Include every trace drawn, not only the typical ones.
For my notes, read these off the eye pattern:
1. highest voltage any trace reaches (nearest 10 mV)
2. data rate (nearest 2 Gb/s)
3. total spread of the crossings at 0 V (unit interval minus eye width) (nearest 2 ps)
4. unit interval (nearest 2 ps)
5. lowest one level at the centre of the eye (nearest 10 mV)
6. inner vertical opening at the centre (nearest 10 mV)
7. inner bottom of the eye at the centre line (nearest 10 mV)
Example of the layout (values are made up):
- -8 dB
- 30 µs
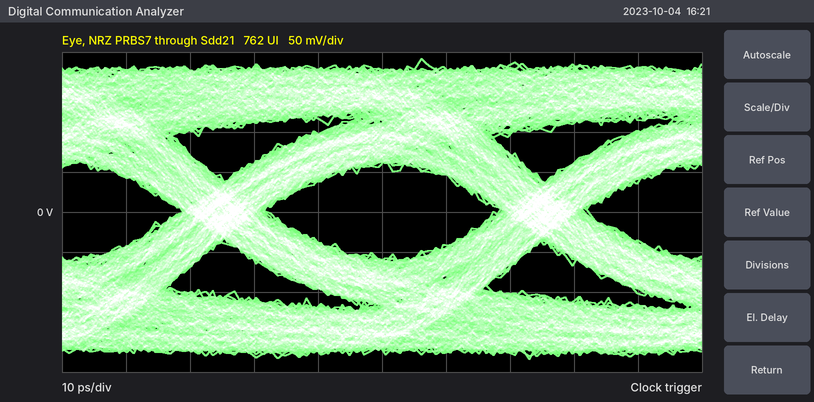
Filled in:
- 190 mV
- 20 Gb/s
- 14 ps
- 50 ps
- 60 mV
- 120 mV
- -60 mV
